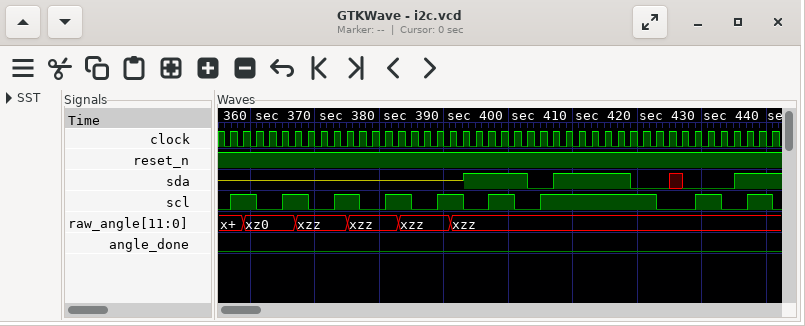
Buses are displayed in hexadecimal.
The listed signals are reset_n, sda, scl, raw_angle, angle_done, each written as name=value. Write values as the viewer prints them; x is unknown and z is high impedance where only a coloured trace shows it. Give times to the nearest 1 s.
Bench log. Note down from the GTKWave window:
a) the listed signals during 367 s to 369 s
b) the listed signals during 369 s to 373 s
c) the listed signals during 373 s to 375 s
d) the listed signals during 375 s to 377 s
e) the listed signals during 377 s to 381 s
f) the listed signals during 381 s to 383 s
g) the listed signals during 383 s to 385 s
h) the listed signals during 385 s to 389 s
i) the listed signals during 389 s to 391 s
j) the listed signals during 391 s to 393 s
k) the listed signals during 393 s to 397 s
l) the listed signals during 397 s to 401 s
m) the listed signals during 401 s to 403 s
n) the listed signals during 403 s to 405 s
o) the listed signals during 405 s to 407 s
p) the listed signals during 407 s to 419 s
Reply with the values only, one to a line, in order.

reset_n=1, sda=z, scl=1, raw_angle=xzz, angle_done=0
reset_n=1, sda=z, scl=0, raw_angle=xzz, angle_done=0
reset_n=1, sda=z, scl=1, raw_angle=xzz, angle_done=0
reset_n=1, sda=z, scl=1, raw_angle=xzz, angle_done=0
reset_n=1, sda=z, scl=0, raw_angle=xzz, angle_done=0
reset_n=1, sda=z, scl=1, raw_angle=xzz, angle_done=0
reset_n=1, sda=z, scl=1, raw_angle=xzz, angle_done=0
reset_n=1, sda=z, scl=0, raw_angle=xzz, angle_done=0
reset_n=1, sda=z, scl=1, raw_angle=xzz, angle_done=0
reset_n=1, sda=z, scl=1, raw_angle=xzz, angle_done=0
reset_n=1, sda=1, scl=0, raw_angle=xzz, angle_done=0
reset_n=1, sda=1, scl=1, raw_angle=xzz, angle_done=0
reset_n=1, sda=1, scl=0, raw_angle=xzz, angle_done=0
reset_n=1, sda=0, scl=0, raw_angle=xzz, angle_done=0
reset_n=1, sda=0, scl=1, raw_angle=xzz, angle_done=0
reset_n=1, sda=1, scl=1, raw_angle=xzz, angle_done=0
